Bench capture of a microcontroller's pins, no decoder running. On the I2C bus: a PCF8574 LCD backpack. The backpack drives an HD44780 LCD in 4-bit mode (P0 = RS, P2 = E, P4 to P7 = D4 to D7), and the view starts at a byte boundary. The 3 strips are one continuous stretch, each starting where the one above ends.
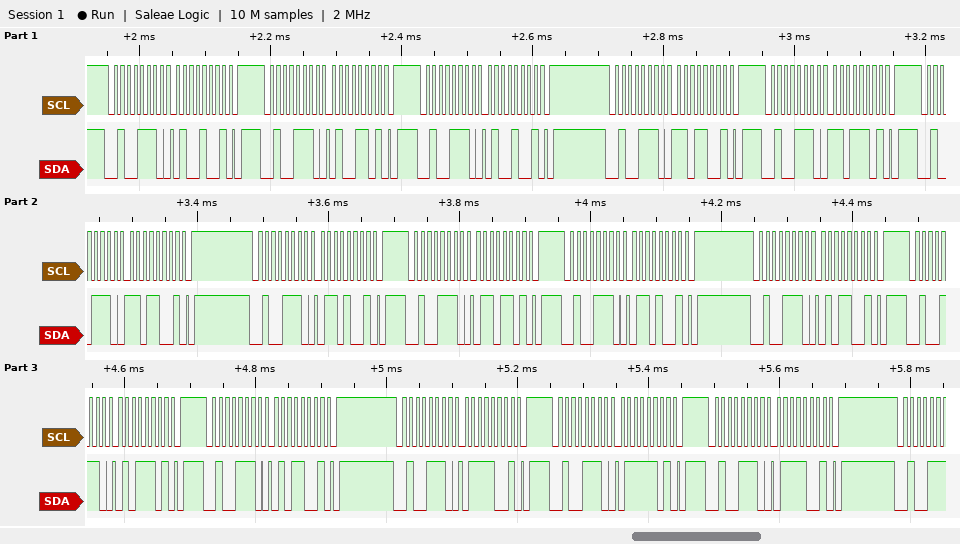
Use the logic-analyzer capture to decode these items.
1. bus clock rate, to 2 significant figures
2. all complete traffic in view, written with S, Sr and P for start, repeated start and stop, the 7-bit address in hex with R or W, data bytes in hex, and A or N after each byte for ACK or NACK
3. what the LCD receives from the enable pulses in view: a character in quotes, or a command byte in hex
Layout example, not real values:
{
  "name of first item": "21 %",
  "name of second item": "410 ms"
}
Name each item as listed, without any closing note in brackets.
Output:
{
  "bus clock rate, to 2 significant figures": "100 kHz",
  "all complete traffic in view, written with S, Sr and P for start, repeated start and stop, the 7-bit address in hex with R or W, data bytes in hex, and A or N after each byte for ACK or NACK": "S 27W A 49 A P S 27W A 4D A P S 27W A 49 A P S 27W A D9 A P S 27W A DD A P S 27W A D9 A P S 27W A 69 A P S 27W A 6D A P S 27W A 69 A P S 27W A 59 A P S 27W A 5D A P S 27W A 59 A P S 27W A 79 A P S 27W A 7D A P S 27W A 79 A P",
  "what the LCD receives from the enable pulses in view: a character in quotes, or a command byte in hex": "'M' 'e'"
}
